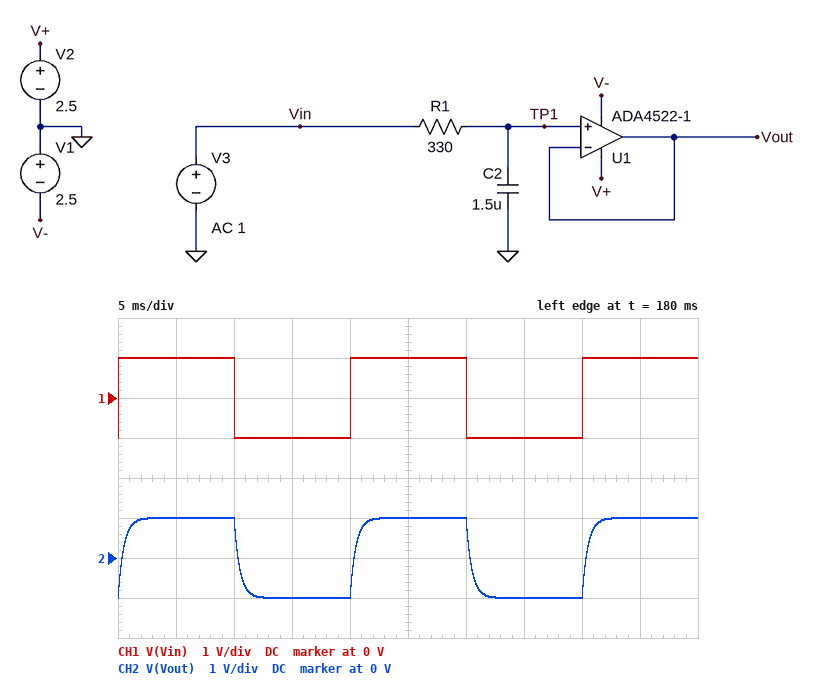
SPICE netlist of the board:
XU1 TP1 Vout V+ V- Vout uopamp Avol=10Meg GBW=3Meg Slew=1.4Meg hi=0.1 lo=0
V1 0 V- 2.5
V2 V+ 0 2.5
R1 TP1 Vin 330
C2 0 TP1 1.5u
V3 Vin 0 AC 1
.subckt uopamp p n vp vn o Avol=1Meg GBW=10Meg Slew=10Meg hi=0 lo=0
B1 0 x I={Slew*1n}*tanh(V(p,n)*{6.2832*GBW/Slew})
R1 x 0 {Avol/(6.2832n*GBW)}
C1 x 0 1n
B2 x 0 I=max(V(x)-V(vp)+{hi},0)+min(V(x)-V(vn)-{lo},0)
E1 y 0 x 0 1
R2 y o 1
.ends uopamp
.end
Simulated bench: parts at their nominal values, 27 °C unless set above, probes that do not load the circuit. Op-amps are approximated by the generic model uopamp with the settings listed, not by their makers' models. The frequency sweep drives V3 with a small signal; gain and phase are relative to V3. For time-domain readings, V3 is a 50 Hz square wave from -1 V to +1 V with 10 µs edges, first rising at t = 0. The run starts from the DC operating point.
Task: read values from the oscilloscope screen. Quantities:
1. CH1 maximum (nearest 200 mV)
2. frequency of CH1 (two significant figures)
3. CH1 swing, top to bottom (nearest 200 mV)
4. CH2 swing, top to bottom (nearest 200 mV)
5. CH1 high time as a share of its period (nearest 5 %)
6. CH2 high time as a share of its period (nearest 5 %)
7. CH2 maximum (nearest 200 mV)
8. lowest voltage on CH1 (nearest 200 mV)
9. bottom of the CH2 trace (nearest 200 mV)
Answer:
1.0 V
50 Hz
2.0 V
2.0 V
50 %
50 %
1.0 V
-1.0 V
-1.0 V
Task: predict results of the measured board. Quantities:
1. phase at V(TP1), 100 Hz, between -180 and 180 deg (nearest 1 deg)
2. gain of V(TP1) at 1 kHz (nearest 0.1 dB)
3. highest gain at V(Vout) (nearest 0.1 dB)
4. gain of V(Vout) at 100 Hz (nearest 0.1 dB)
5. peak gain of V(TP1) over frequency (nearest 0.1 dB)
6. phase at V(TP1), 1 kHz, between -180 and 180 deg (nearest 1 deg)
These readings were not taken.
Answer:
-17 deg
-10.3 dB
0 dB
-0.4 dB
0 dB
-72 deg
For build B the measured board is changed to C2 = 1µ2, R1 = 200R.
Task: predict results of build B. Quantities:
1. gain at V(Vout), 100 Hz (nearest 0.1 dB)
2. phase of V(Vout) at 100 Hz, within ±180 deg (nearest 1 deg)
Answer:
-0.1 dB
-9 deg
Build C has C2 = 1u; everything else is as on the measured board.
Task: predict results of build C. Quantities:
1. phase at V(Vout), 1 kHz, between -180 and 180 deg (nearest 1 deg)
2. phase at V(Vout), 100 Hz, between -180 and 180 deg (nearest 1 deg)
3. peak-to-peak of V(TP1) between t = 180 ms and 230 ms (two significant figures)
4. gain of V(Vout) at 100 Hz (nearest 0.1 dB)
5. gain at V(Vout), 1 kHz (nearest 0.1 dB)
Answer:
-64 deg
-12 deg
2.0 V
-0.2 dB
-7.2 dB
